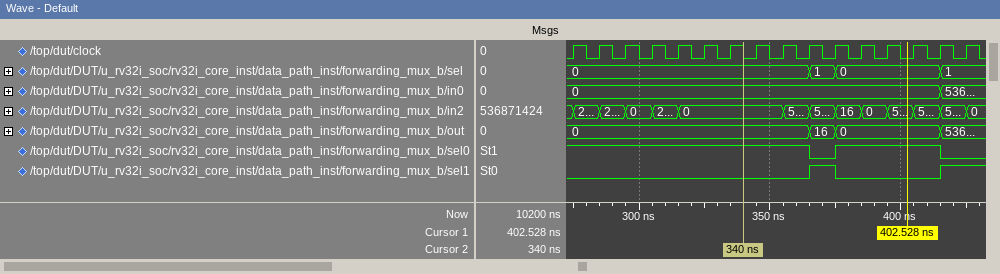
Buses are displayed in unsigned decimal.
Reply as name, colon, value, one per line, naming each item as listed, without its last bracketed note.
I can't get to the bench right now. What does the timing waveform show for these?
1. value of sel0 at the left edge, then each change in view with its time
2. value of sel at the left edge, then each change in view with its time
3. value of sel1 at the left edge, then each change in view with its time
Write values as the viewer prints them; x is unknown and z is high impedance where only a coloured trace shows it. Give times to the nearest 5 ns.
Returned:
value of sel0 at the left edge, then each change in view with its time: 1, 0 at 365 ns, 1 at 375 ns, 0 at 415 ns
value of sel at the left edge, then each change in view with its time: 0, 1 at 365 ns, 0 at 375 ns, 1 at 415 ns
value of sel1 at the left edge, then each change in view with its time: 0, 1 at 365 ns, 0 at 375 ns, 1 at 415 ns
